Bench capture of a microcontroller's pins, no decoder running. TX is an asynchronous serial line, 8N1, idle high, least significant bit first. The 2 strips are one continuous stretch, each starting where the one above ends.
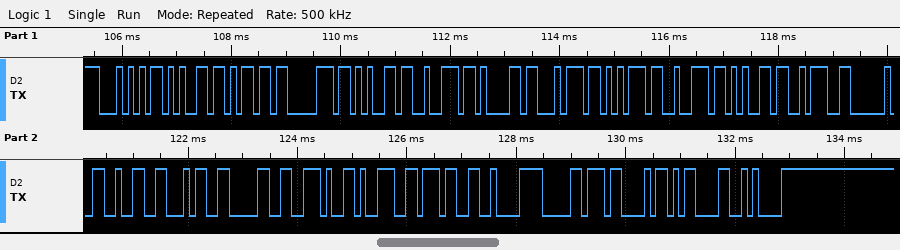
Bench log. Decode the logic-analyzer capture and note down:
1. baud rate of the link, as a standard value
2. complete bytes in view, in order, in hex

9600 baud
54 65 6D 70 65 72 61 74 75 72 65 3A 20 32 34 30 2E 39 37 C2 B0 43 0D 0A
